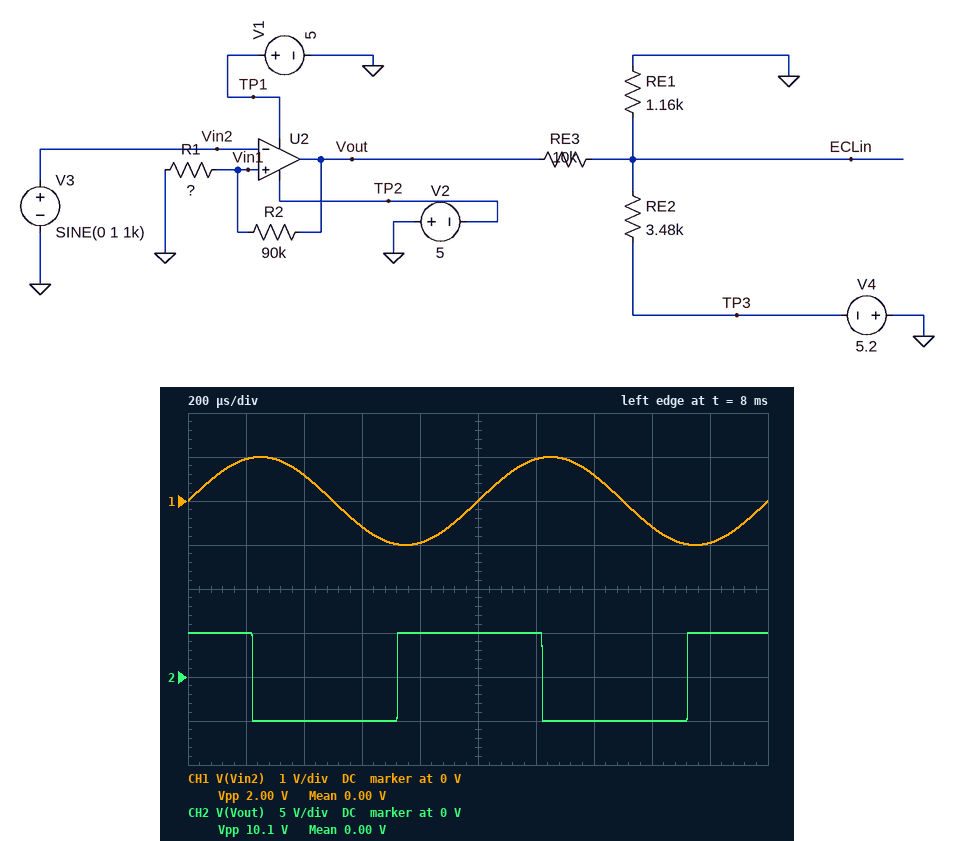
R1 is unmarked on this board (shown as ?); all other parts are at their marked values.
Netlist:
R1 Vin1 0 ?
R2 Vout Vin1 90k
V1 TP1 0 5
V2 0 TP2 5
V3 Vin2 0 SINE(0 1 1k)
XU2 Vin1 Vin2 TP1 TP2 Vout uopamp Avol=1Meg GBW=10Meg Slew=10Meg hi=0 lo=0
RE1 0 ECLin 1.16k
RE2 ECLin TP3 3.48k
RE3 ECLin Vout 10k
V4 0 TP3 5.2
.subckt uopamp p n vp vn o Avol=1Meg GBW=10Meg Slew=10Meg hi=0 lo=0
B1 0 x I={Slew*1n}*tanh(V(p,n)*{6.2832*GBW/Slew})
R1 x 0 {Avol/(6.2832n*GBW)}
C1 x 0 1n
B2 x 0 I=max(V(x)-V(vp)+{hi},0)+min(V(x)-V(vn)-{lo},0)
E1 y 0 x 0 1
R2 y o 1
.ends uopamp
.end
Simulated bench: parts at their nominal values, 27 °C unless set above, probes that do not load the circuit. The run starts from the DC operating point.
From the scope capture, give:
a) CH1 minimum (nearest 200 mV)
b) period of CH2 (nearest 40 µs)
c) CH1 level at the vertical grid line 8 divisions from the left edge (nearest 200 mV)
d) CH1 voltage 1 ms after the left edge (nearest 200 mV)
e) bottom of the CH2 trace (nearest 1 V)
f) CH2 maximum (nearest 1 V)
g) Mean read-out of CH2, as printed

-1.0 V
1.00 ms
-600 mV
0 V
-5 V
5 V
0.00 V
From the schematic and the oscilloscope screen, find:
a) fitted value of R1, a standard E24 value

22 kΩ
